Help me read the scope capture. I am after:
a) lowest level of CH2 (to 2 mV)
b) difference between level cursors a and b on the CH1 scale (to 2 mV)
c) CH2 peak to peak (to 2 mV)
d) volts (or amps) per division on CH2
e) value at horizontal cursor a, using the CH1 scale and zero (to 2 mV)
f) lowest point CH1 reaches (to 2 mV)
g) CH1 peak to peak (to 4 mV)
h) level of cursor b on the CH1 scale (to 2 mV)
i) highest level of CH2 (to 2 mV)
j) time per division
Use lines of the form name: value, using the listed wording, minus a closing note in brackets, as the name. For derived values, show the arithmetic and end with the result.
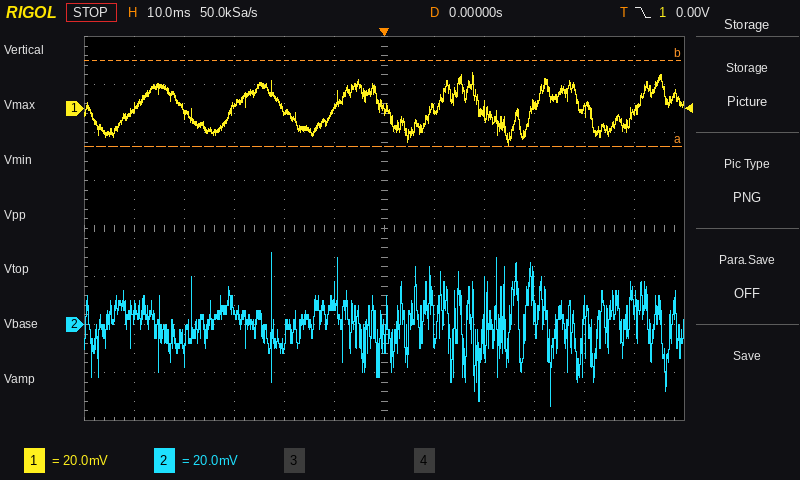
lowest level of CH2: -34 mV
difference between level cursors a and b on the CH1 scale: 36 mV
CH2 peak to peak: 30 mV − (-34 mV) = 64 mV
volts (or amps) per division on CH2: 20 mV
value at horizontal cursor a, using the CH1 scale and zero: -16 mV
lowest point CH1 reaches: -16 mV
CH1 peak to peak: 32 mV
level of cursor b on the CH1 scale: 20 mV
highest level of CH2: 30 mV
time per division: 10 ms
